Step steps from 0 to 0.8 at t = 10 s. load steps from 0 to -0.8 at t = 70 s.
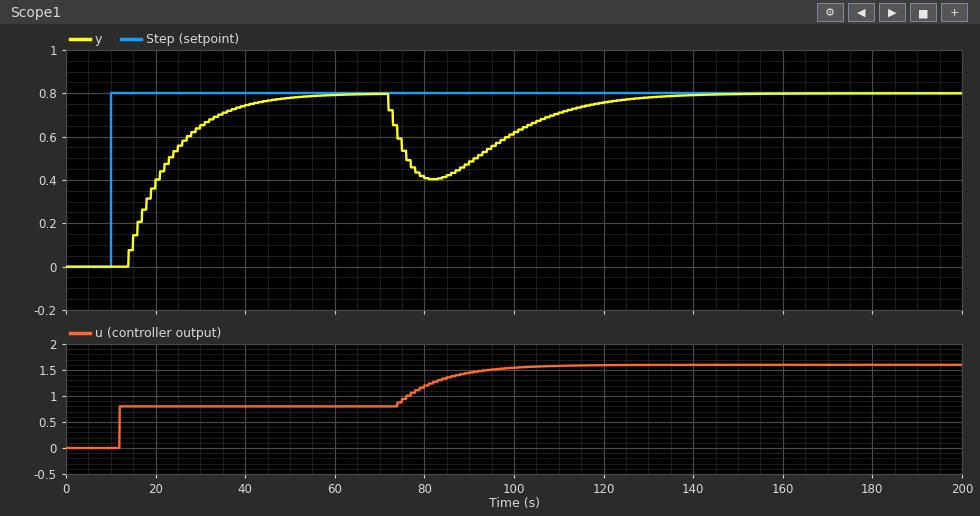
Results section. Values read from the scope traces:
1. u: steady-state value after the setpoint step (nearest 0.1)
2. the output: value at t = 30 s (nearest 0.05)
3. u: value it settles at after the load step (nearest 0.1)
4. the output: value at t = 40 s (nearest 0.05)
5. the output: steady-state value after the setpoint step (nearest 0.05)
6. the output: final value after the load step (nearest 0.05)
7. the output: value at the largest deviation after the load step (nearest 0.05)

0.8
0.65
1.6
0.75
0.80
0.80
0.40
